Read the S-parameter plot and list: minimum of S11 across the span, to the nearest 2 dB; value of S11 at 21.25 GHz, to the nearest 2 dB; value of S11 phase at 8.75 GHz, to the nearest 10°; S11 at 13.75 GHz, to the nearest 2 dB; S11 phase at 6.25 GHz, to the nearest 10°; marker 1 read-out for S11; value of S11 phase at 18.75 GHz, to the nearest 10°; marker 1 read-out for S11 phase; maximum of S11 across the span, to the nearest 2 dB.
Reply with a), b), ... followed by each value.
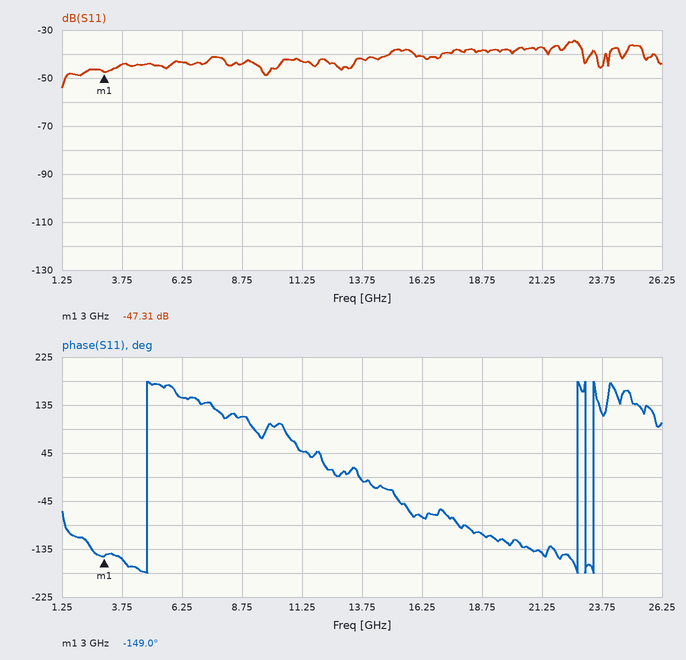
a) -54 dB
b) -38 dB
c) 110°
d) -42 dB
e) 150°
f) -47.31 dB
g) -110°
h) -149.0°
i) -34 dB
